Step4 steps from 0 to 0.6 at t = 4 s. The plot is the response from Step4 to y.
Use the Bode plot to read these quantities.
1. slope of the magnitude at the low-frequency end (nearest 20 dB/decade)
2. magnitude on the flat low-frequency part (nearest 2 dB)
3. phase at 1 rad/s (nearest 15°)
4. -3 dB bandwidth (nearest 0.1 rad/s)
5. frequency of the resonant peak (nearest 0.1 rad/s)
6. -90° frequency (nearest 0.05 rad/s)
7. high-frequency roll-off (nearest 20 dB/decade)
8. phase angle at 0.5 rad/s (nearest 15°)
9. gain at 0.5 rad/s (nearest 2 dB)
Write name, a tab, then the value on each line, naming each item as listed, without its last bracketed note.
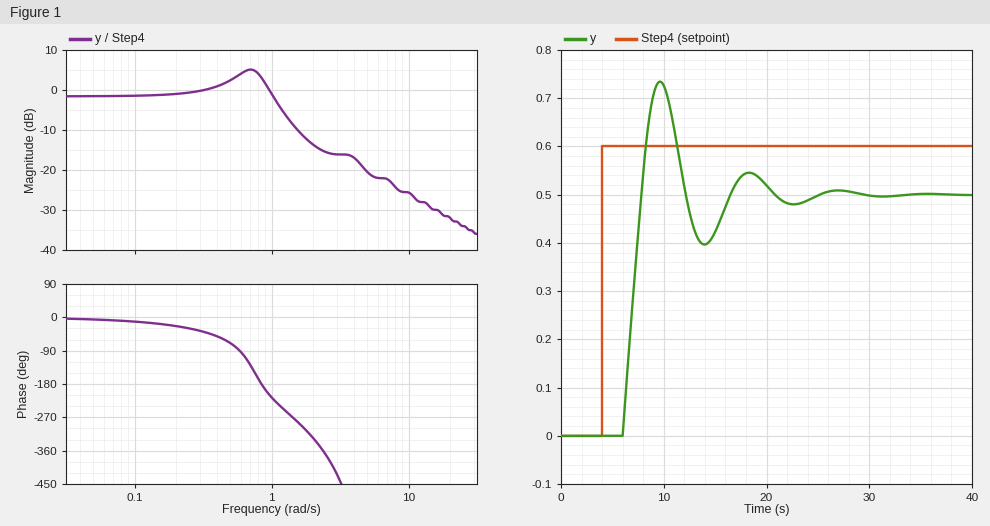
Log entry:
slope of the magnitude at the low-frequency end	0 dB/decade
magnitude on the flat low-frequency part	-2 dB
phase at 1 rad/s	-210°
-3 dB bandwidth	1.2 rad/s
frequency of the resonant peak	0.7 rad/s
-90° frequency	0.60 rad/s
high-frequency roll-off	-20 dB/decade
phase angle at 0.5 rad/s	-75°
gain at 0.5 rad/s	2 dB
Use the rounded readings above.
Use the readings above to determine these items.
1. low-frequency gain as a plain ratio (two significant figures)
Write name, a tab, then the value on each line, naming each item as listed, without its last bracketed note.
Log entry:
low-frequency gain as a plain ratio	0.79
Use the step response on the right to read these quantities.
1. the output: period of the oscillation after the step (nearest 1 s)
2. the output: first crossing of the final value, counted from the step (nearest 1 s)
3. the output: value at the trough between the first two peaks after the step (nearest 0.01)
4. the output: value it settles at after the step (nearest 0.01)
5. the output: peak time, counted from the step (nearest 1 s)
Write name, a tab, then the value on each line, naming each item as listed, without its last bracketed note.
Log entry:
the output: period of the oscillation after the step	9 s
the output: first crossing of the final value, counted from the step	4 s
the output: value at the trough between the first two peaks after the step	0.40
the output: value it settles at after the step	0.50
the output: peak time, counted from the step	6 s
